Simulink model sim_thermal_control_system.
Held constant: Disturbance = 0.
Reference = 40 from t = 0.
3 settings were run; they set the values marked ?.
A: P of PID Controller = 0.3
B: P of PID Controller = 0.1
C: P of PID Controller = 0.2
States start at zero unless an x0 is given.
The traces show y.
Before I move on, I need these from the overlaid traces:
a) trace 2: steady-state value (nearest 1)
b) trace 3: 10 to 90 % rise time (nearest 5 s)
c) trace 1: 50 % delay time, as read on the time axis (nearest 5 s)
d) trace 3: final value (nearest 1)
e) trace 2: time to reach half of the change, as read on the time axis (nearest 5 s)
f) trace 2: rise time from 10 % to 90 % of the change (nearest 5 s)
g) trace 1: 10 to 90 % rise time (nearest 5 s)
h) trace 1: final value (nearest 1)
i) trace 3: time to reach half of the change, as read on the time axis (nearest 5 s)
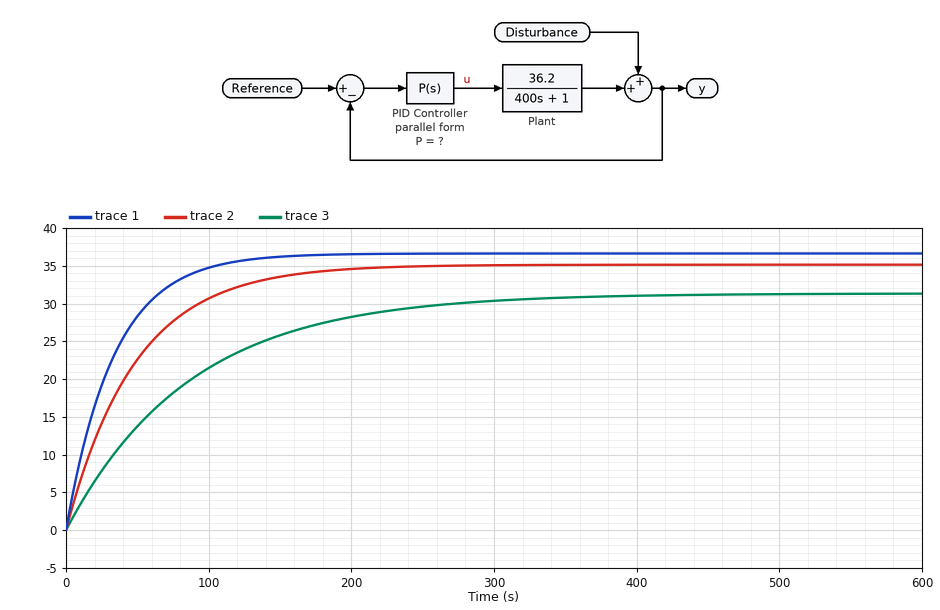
35
190 s
25 s
31
35 s
105 s
75 s
37
60 s
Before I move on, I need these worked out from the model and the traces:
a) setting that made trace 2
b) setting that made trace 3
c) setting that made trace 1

C
B
A
